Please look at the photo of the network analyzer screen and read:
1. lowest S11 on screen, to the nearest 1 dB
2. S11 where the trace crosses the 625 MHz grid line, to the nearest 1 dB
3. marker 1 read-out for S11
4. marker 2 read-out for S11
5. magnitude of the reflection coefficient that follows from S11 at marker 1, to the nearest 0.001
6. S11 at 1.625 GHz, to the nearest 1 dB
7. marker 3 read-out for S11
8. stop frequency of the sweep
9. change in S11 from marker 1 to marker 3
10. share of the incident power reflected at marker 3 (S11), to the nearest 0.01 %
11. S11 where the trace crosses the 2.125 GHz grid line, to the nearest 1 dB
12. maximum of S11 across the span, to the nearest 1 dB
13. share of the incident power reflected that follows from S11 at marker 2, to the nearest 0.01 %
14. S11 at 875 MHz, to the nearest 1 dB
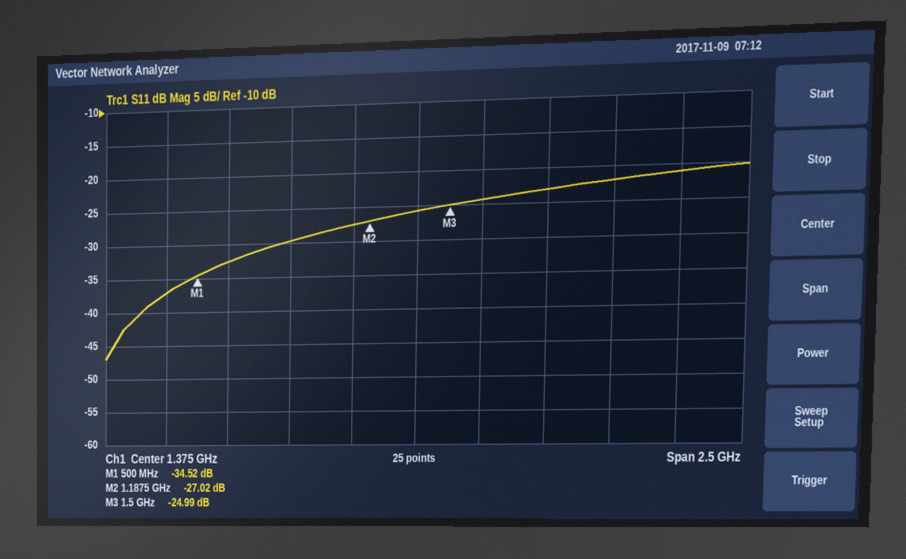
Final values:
-47 dB
-33 dB
-34.52 dB
-27.02 dB
0.019
-24 dB
-24.99 dB
2.625 GHz
9.53 dB
0.32 %
-22 dB
-20 dB
0.20 %
-30 dB
